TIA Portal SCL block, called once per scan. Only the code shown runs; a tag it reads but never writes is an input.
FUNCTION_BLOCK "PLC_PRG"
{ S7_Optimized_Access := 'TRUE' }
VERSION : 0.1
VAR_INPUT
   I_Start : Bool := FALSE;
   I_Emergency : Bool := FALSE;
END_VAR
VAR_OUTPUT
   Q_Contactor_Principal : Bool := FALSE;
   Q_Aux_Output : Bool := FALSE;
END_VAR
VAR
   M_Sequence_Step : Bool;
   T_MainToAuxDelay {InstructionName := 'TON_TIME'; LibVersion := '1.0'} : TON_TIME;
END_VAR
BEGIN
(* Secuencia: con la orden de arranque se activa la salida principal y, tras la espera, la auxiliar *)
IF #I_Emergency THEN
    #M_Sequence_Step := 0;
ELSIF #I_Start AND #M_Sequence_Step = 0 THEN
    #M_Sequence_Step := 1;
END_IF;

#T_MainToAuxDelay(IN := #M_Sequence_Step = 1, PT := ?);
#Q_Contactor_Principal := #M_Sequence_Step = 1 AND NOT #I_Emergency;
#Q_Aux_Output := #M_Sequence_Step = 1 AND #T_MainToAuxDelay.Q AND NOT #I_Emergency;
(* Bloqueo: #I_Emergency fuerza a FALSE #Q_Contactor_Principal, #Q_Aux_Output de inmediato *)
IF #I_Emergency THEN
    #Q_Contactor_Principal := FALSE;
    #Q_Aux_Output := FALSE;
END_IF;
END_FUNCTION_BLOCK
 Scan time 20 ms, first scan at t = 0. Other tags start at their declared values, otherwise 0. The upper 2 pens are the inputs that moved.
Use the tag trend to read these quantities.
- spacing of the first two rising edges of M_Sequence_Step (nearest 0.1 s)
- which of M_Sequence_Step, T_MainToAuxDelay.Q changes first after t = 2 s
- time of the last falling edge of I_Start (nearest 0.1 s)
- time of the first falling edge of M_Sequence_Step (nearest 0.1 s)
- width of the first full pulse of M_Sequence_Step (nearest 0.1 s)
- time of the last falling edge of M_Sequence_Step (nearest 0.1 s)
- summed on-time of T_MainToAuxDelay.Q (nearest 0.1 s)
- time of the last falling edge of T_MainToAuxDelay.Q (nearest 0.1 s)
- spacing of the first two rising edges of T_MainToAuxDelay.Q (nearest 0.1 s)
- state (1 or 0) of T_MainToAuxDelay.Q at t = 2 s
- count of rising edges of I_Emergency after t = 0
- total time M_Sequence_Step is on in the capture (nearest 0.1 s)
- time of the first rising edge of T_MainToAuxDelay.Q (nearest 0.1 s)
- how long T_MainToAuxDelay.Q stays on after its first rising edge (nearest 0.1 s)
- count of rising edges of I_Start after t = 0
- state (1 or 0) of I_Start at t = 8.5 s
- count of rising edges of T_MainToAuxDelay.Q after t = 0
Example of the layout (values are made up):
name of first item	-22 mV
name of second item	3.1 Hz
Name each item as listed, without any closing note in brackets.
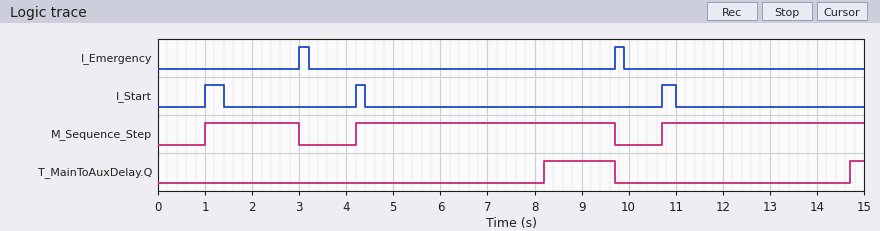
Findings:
spacing of the first two rising edges of M_Sequence_Step	3.2 s
which of M_Sequence_Step, T_MainToAuxDelay.Q changes first after t = 2 s	M_Sequence_Step
time of the last falling edge of I_Start	11.0 s
time of the first falling edge of M_Sequence_Step	3.0 s
width of the first full pulse of M_Sequence_Step	2.0 s
time of the last falling edge of M_Sequence_Step	9.7 s
summed on-time of T_MainToAuxDelay.Q	1.8 s
time of the last falling edge of T_MainToAuxDelay.Q	9.7 s
spacing of the first two rising edges of T_MainToAuxDelay.Q	6.5 s
state (1 or 0) of T_MainToAuxDelay.Q at t = 2 s	0
count of rising edges of I_Emergency after t = 0	2
total time M_Sequence_Step is on in the capture	11.8 s
time of the first rising edge of T_MainToAuxDelay.Q	8.2 s
how long T_MainToAuxDelay.Q stays on after its first rising edge	1.5 s
count of rising edges of I_Start after t = 0	3
state (1 or 0) of I_Start at t = 8.5 s	0
count of rising edges of T_MainToAuxDelay.Q after t = 0	2
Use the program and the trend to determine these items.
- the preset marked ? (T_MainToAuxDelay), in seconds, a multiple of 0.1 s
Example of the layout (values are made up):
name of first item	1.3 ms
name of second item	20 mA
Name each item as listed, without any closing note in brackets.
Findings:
the preset marked ? (T_MainToAuxDelay), in seconds, a multiple of 0.1 s	4.0 s
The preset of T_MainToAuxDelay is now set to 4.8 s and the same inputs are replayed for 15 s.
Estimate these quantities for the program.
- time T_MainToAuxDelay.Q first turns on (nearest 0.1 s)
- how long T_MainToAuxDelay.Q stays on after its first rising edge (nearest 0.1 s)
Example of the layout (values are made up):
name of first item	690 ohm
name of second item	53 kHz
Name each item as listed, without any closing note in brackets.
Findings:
time T_MainToAuxDelay.Q first turns on	9.0 s
how long T_MainToAuxDelay.Q stays on after its first rising edge	0.7 s
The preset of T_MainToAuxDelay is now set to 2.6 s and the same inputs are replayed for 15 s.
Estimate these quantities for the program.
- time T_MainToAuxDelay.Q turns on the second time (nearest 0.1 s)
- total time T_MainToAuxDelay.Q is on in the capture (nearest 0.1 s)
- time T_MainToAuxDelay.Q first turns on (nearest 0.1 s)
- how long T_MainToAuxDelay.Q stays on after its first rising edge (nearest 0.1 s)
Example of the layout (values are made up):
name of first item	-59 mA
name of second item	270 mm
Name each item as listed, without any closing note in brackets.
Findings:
time T_MainToAuxDelay.Q turns on the second time	13.3 s
total time T_MainToAuxDelay.Q is on in the capture	4.6 s
time T_MainToAuxDelay.Q first turns on	6.8 s
how long T_MainToAuxDelay.Q stays on after its first rising edge	2.9 s
